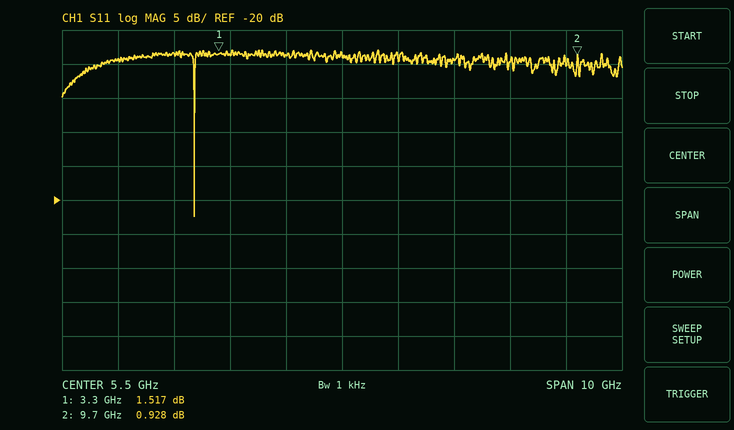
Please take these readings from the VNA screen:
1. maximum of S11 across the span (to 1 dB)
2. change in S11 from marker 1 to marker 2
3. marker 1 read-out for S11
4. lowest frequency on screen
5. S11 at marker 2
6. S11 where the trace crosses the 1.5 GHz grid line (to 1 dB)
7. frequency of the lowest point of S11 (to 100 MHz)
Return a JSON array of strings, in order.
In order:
["2 dB", "-0.589 dB", "1.517 dB", "500 MHz", "0.928 dB", "1 dB", "2.9 GHz"]
